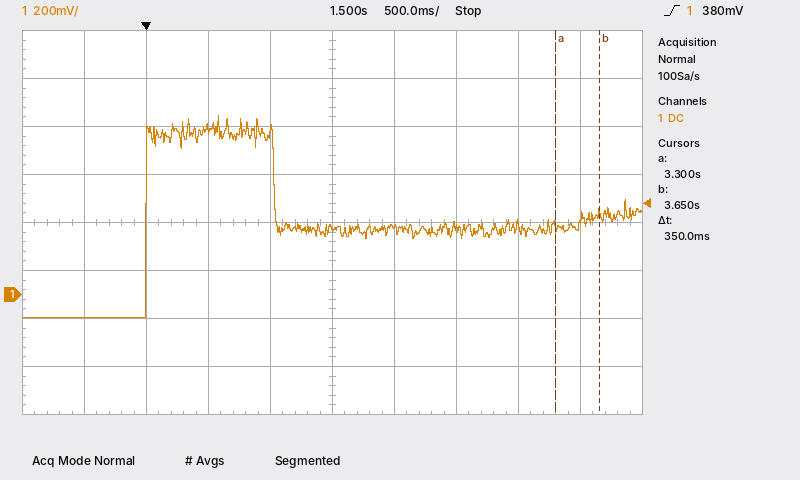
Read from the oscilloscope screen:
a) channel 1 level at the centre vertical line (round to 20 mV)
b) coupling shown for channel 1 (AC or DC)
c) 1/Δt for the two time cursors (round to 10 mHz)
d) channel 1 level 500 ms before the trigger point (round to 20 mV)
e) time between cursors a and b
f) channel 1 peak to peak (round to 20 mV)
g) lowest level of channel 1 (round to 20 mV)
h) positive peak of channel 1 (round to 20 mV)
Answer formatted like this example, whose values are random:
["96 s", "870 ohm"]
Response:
["280 mV", "DC", "2.86 Hz", "-100 mV", "350 ms", "840 mV", "-100 mV", "740 mV"]
